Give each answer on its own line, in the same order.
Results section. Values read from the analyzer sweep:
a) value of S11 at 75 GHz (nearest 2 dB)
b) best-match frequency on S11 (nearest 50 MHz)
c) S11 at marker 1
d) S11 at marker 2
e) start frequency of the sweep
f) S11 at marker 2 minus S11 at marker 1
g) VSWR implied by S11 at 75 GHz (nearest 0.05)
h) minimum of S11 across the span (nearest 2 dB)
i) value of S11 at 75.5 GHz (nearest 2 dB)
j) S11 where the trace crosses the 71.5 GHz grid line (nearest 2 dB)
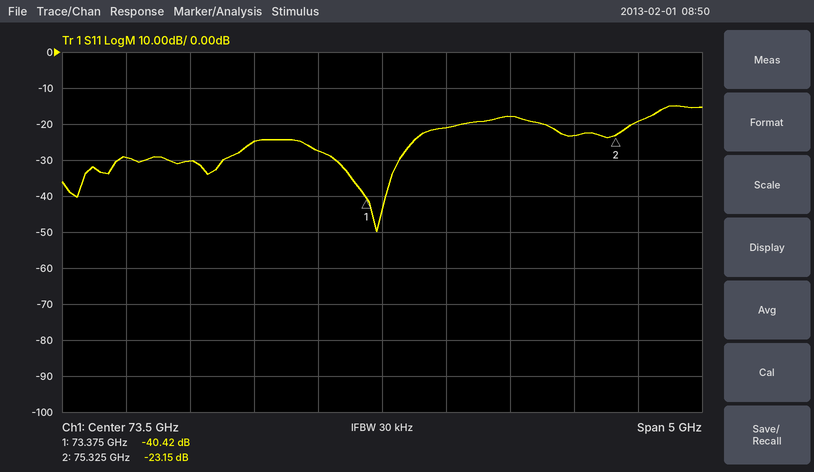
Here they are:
-24 dB
73.45 GHz
-40.42 dB
-23.15 dB
71 GHz
17.27 dB
1.15
-50 dB
-20 dB
-30 dB
